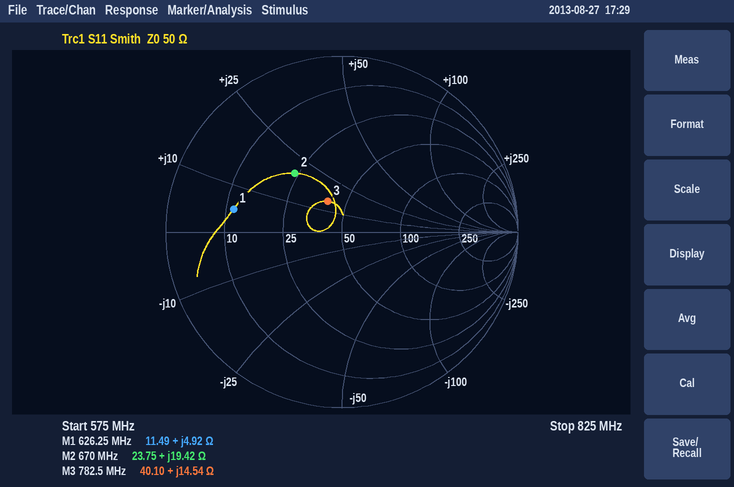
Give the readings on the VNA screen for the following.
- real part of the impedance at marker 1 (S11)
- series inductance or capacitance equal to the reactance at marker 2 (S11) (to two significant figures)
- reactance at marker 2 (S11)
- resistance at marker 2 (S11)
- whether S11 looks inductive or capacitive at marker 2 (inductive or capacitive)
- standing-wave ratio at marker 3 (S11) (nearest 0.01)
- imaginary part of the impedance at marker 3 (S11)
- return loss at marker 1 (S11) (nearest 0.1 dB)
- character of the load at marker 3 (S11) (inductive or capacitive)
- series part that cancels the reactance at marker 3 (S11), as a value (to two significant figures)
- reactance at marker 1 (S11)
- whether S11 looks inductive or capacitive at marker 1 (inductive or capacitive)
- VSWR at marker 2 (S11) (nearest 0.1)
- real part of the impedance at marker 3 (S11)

11.49 Ω
4.6 nH
+19.42 Ω
23.75 Ω
inductive
1.48
+14.54 Ω
4.0 dB
inductive
14 pF
+4.92 Ω
inductive
2.5
40.10 Ω
